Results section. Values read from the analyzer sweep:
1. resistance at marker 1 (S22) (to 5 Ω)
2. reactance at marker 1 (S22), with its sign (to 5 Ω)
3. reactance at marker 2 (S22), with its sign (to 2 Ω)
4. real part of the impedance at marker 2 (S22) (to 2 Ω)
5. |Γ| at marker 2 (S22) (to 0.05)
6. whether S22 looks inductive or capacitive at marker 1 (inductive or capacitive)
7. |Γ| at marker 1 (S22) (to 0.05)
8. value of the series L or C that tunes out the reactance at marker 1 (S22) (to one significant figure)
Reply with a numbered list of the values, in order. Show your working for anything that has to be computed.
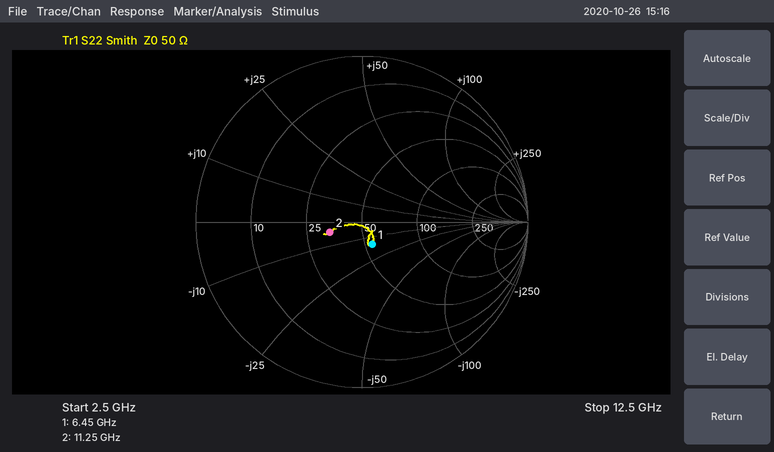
1. 55 Ω
2. -15 Ω
3. -4 Ω
4. 34 Ω
5. 0.20
6. capacitive
7. 0.15
8. L = 15 Ω/(2π × 6.45 GHz) ≈ 370 pH, so 400 pH to one significant figure
